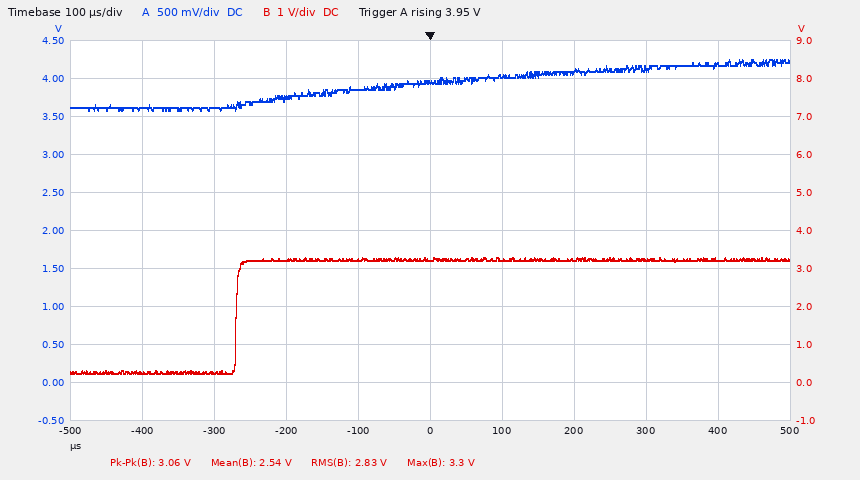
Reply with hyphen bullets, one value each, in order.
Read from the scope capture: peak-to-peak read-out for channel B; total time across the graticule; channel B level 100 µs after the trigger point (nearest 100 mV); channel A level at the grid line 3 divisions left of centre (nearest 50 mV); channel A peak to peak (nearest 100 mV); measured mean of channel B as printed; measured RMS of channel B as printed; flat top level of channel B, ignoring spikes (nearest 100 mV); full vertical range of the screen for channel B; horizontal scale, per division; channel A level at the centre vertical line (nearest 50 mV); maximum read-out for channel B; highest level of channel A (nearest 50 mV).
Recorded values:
- 3.06 V
- 1 ms
- 3.2 V
- 3.60 V
- 700 mV
- 2.54 V
- 2.83 V
- 3.2 V
- 10 V
- 100 µs
- 3.95 V
- 3.3 V
- 4.25 V
